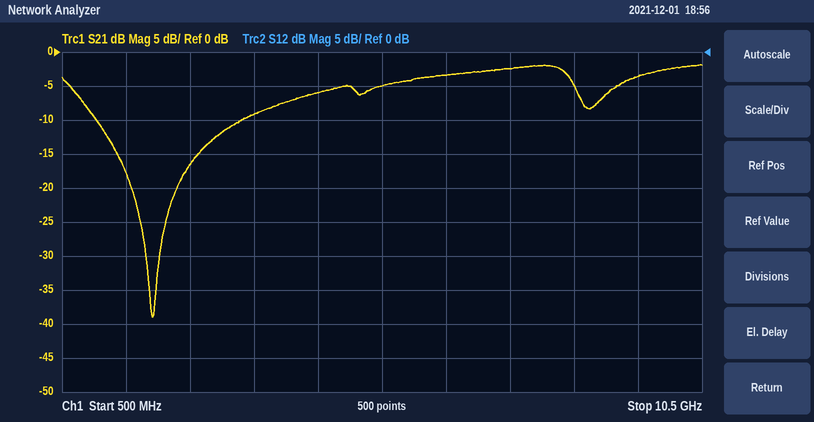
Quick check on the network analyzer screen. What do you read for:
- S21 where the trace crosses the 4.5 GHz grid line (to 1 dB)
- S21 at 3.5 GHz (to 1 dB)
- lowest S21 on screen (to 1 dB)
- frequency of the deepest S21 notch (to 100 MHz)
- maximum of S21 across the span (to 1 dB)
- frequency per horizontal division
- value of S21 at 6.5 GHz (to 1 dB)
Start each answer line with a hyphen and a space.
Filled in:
- -6 dB
- -9 dB
- -39 dB
- 1.9 GHz
- -2 dB
- 1 GHz
- -3 dB
